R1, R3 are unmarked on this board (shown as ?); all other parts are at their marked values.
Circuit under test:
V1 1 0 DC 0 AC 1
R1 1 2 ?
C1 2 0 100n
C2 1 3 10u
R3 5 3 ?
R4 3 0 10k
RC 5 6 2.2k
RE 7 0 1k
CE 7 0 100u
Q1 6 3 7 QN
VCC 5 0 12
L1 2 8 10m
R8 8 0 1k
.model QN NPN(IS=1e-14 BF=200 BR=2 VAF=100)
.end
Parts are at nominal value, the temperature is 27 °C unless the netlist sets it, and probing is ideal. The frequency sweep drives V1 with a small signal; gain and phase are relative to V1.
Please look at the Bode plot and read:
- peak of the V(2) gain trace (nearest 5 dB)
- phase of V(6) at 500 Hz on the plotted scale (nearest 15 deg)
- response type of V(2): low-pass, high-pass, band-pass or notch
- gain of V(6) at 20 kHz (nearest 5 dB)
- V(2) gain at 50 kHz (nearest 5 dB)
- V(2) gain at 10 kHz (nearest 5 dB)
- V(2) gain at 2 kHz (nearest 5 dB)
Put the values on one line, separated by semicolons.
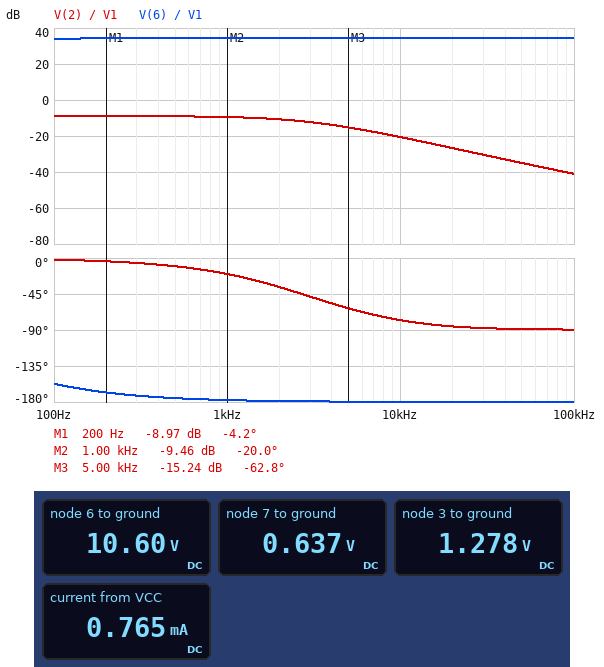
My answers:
-10 dB; -180 deg; low-pass; 35 dB; -35 dB; -20 dB; -10 dB
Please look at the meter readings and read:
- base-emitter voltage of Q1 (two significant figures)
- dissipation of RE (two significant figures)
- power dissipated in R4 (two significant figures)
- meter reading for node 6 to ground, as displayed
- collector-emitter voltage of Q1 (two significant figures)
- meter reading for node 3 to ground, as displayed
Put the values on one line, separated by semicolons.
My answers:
640 mV; 410 µW; 160 µW; 10.60 V; 10 V; 1.278 V
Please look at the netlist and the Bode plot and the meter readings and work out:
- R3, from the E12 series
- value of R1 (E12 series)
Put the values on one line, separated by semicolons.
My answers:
82 kΩ; 1.8 kΩ
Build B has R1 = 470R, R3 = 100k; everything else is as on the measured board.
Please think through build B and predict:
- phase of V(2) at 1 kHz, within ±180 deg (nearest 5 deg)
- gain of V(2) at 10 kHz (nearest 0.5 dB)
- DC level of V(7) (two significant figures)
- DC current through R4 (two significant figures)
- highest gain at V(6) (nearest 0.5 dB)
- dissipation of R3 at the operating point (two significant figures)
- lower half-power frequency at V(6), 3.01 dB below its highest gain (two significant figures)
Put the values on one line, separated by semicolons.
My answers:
-10 deg; -9.5 dB; 440 mV; 110 µA; 31.5 dB; 1.2 mW; 30 Hz
